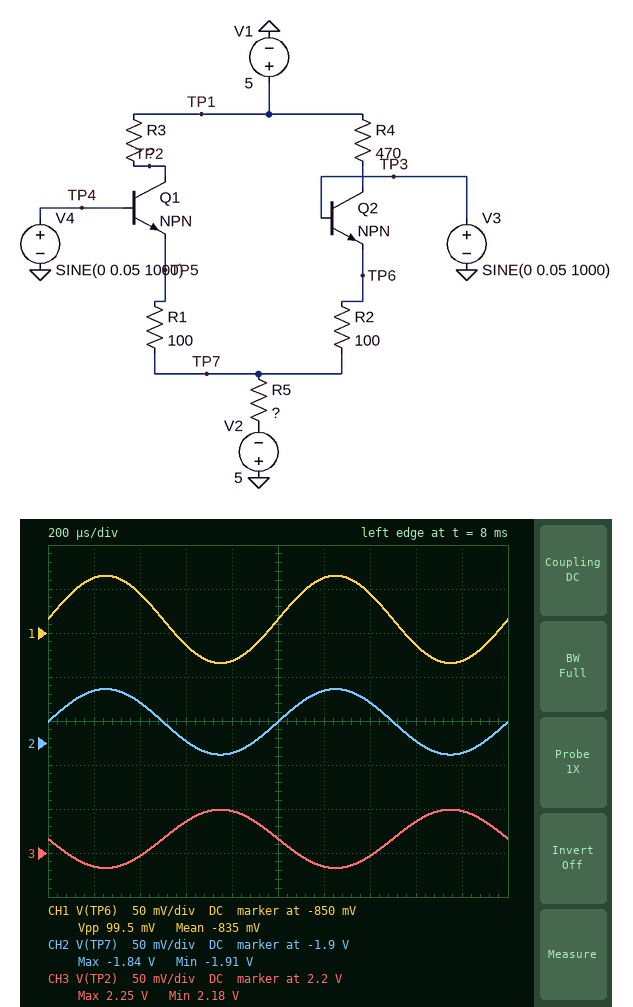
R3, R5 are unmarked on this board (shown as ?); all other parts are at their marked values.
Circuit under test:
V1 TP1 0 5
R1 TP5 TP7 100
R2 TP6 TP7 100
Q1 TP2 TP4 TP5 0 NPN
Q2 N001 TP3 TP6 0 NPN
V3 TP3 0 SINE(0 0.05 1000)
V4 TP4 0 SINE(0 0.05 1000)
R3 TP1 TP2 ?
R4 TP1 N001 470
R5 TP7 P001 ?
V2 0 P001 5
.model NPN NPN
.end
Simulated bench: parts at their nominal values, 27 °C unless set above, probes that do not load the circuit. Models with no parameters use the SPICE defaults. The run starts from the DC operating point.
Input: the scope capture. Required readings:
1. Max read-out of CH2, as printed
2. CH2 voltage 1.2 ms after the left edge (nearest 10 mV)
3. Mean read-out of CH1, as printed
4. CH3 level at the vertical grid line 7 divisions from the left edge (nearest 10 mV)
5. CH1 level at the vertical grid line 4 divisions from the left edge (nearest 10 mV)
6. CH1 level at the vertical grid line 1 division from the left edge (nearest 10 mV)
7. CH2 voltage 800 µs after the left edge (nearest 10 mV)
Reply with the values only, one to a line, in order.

-1.84 V
-1.84 V
-835 mV
2.20 V
-880 mV
-790 mV
-1.91 V
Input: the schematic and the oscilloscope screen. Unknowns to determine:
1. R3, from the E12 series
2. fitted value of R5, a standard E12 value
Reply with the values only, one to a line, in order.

270 Ω
150 Ω
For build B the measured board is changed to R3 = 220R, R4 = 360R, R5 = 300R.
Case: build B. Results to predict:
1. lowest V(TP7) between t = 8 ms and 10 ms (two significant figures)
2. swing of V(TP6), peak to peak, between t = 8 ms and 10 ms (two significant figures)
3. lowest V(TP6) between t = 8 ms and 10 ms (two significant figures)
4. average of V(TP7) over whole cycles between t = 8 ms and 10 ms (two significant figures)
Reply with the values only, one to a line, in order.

-1.5 V
99 mV
-870 mV
-1.4 V
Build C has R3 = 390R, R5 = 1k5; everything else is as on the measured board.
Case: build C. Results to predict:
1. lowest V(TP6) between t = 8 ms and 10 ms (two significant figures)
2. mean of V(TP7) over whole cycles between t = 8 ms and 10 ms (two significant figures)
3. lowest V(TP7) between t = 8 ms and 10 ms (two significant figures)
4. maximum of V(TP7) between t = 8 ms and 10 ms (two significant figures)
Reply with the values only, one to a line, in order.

-830 mV
-920 mV
-970 mV
-870 mV
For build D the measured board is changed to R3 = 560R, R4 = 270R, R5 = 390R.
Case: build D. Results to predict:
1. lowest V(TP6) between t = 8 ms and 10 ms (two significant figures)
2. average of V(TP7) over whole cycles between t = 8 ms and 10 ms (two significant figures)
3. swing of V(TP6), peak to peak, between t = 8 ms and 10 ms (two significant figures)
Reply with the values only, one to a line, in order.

-860 mV
-1.3 V
99 mV
